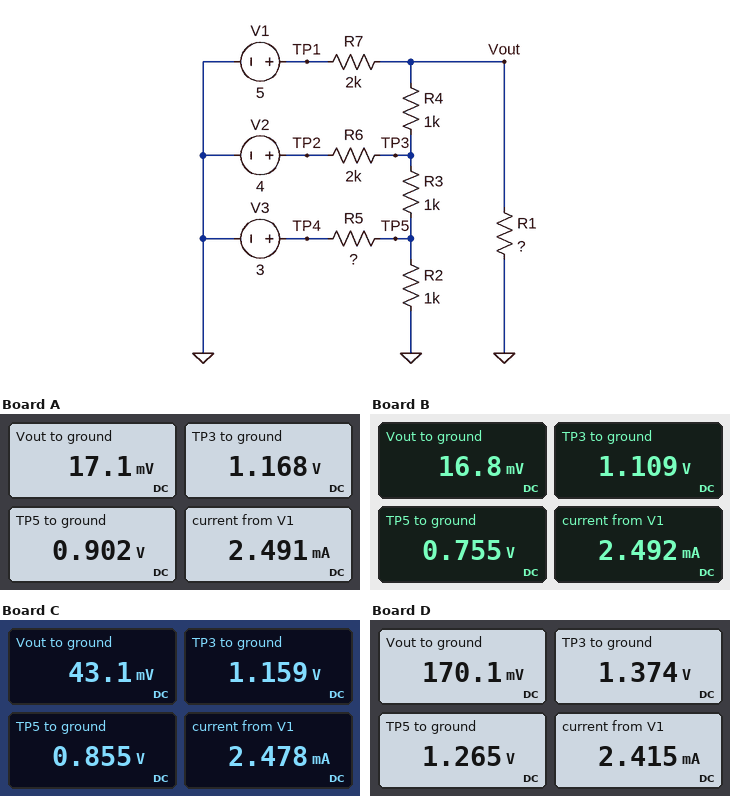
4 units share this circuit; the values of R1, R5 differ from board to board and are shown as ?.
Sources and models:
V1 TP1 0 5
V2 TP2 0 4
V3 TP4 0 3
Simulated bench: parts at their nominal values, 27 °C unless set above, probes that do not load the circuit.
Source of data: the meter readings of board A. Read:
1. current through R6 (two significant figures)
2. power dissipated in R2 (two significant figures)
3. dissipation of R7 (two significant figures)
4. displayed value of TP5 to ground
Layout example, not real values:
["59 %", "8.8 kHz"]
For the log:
["1.4 mA", "810 µW", "12 mW", "0.902 V"]
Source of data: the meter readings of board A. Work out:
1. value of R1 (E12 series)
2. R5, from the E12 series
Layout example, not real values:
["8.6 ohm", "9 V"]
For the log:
["4.7 Ω", "3.3 kΩ"]
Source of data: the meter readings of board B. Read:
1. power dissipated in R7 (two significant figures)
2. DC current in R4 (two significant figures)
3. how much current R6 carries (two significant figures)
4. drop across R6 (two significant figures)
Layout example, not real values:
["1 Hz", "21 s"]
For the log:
["12 mW", "1.1 mA", "1.4 mA", "2.9 V"]
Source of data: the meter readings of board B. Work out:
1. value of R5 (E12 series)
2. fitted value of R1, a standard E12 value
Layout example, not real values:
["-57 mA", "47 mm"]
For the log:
["5.6 kΩ", "4.7 Ω"]
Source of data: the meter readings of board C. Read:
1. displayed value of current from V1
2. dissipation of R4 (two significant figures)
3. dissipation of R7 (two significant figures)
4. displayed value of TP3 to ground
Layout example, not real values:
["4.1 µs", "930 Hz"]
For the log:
["2.478 mA", "1.2 mW", "12 mW", "1.159 V"]
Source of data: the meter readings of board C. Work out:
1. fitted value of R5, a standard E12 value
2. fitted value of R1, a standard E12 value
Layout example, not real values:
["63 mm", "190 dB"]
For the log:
["3.9 kΩ", "12 Ω"]
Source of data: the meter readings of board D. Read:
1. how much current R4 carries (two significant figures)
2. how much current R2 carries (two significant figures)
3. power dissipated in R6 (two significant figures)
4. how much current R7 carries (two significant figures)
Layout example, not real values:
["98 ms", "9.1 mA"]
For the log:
["1.2 mA", "1.3 mA", "3.4 mW", "2.4 mA"]
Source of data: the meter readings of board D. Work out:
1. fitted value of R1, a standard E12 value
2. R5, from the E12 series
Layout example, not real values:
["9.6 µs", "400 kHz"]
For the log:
["47 Ω", "1.5 kΩ"]
